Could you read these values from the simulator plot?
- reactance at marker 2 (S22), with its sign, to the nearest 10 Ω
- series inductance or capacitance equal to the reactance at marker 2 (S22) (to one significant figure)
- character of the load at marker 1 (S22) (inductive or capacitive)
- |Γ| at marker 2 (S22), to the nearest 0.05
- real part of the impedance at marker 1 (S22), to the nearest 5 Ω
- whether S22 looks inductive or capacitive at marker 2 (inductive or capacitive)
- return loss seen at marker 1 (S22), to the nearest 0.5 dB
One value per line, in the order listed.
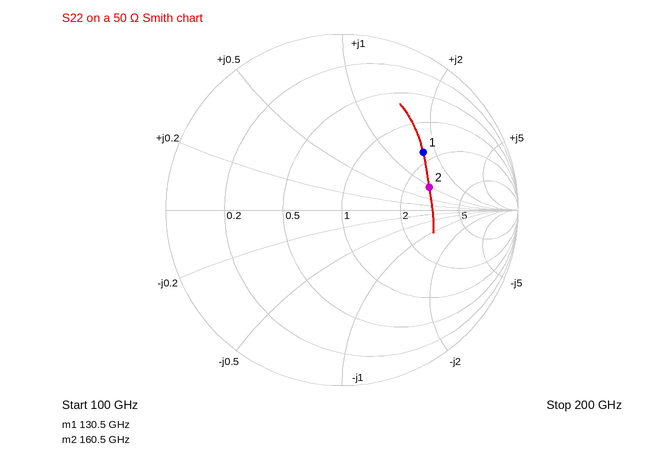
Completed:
+50 Ω
50 pH
inductive
0.50
85 Ω
inductive
5.0 dB
